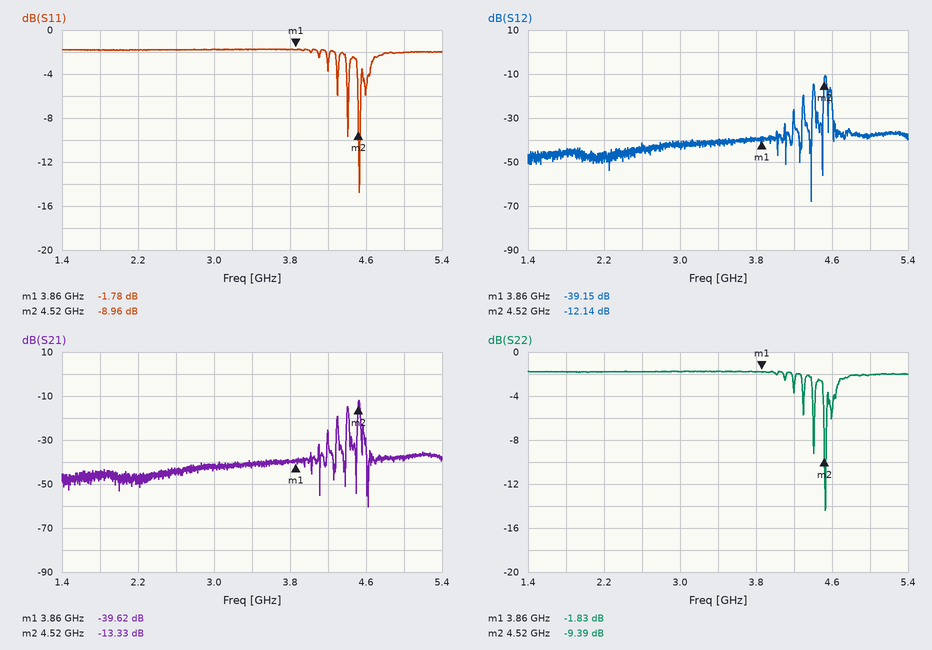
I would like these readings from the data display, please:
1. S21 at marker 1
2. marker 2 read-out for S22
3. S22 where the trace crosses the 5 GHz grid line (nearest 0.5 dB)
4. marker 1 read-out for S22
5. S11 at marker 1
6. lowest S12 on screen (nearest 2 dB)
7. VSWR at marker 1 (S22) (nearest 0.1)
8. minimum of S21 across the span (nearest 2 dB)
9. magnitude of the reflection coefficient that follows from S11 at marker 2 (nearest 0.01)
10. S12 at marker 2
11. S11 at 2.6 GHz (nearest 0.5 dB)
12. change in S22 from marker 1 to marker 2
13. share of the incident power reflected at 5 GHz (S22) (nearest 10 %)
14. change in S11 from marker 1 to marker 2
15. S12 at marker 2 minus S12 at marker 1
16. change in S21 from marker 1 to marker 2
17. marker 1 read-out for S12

-39.62 dB
-9.39 dB
-2.0 dB
-1.83 dB
-1.78 dB
-68 dB
9.5
-60 dB
0.36
-12.14 dB
-2.0 dB
-7.56 dB
60 %
-7.18 dB
27.01 dB
26.29 dB
-39.15 dB
